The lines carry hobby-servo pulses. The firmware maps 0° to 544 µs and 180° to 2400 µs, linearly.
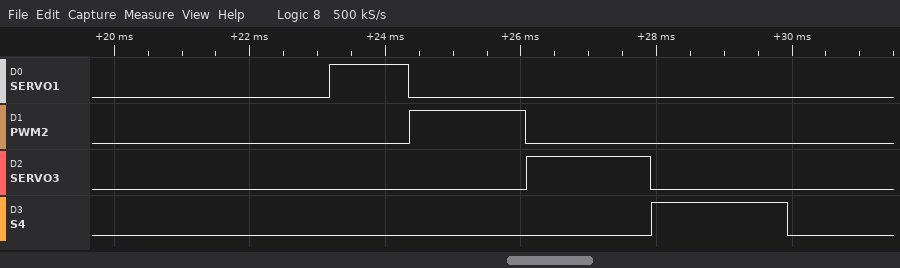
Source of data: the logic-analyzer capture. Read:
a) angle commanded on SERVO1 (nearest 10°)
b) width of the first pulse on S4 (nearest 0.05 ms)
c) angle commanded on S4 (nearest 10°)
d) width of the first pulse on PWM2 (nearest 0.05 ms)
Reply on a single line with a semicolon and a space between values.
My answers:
60°; 2.00 ms; 140°; 1.70 ms
